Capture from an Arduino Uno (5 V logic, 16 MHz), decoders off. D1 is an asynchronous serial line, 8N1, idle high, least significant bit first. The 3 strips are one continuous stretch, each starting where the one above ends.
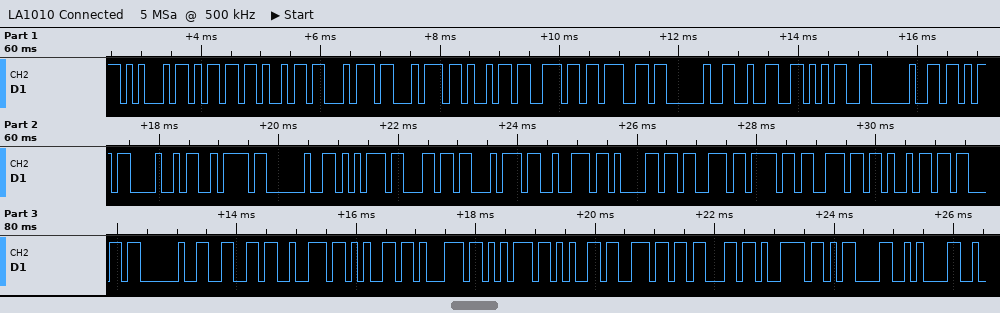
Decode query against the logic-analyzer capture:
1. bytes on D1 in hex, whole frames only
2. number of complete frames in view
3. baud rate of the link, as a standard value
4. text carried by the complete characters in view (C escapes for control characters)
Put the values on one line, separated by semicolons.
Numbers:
45 6D 69 74 74 69 6E 67 20 32 35 20 6B 48 7A 20 75 6C 74 72 61 73 6F 6E 69 63 20 66 72 65 71 75 65 6E 63 79 0D 0A; 38; 9600 baud; "Emitting 25 kHz ultrasonic frequency\r\n"
